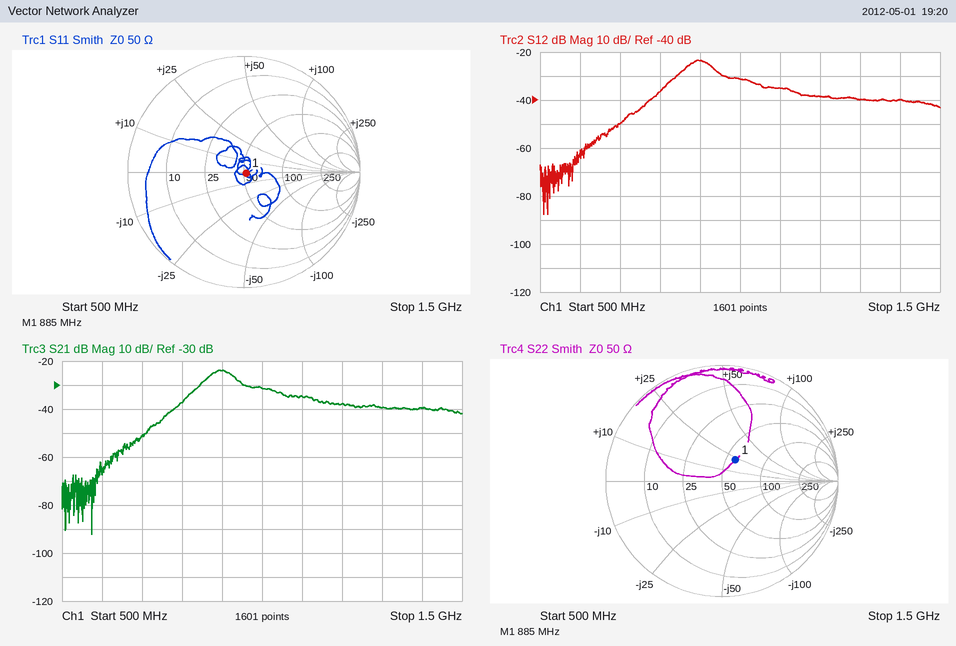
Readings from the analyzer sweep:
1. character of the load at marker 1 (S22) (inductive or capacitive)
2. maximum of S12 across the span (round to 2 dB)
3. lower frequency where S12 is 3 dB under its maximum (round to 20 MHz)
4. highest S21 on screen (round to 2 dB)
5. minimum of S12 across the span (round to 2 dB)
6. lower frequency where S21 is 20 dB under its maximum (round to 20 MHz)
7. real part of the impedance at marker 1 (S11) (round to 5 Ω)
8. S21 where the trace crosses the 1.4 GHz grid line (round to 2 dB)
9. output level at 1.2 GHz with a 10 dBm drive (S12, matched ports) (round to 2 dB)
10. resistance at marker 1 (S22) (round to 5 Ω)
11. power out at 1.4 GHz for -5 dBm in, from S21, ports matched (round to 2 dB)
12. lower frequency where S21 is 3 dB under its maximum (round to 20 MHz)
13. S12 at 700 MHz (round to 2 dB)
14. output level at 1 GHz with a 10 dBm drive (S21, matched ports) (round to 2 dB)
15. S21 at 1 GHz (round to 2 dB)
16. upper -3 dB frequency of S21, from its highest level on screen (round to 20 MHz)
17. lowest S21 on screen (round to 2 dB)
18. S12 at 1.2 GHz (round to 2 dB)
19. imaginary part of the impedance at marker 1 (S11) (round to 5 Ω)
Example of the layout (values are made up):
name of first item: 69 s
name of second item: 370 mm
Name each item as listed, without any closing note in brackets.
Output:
character of the load at marker 1 (S22): inductive
maximum of S12 across the span: -24 dB
lower frequency where S12 is 3 dB under its maximum: 860 MHz
highest S21 on screen: -24 dB
minimum of S12 across the span: -88 dB
lower frequency where S21 is 20 dB under its maximum: 760 MHz
real part of the impedance at marker 1 (S11): 50 Ω
S21 where the trace crosses the 1.4 GHz grid line: -40 dB
output level at 1.2 GHz with a 10 dBm drive (S12, matched ports): -28 dBm
resistance at marker 1 (S22): 60 Ω
power out at 1.4 GHz for -5 dBm in, from S21, ports matched: -44 dBm
lower frequency where S21 is 3 dB under its maximum: 860 MHz
S12 at 700 MHz: -50 dB
output level at 1 GHz with a 10 dBm drive (S21, matched ports): -22 dBm
S21 at 1 GHz: -32 dB
upper -3 dB frequency of S21, from its highest level on screen: 940 MHz
lowest S21 on screen: -92 dB
S12 at 1.2 GHz: -38 dB
imaginary part of the impedance at marker 1 (S11): 0 Ω
